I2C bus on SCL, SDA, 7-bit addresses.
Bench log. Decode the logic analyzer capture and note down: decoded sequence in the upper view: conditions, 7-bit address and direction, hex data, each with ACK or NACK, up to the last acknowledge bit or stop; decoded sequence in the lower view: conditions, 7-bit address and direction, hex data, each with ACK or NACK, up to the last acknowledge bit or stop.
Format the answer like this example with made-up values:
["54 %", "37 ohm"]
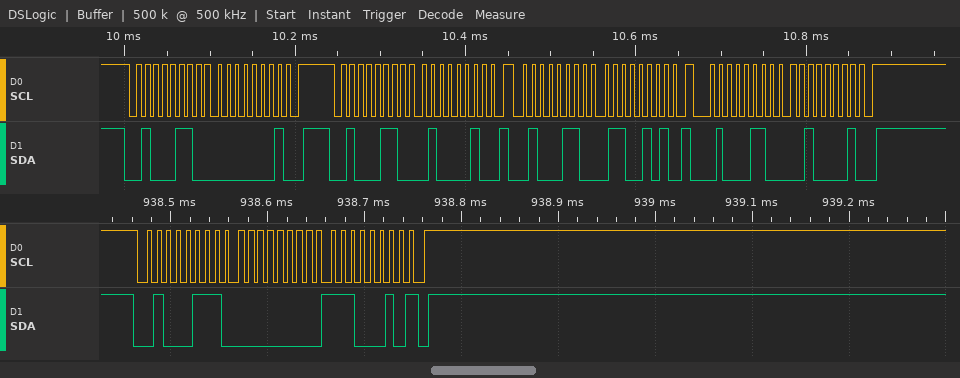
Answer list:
["start, address 23 write ACK, 01 ACK, stop, start, address 23 write ACK, 42 ACK, repeated start, address 23 write ACK, 65 ACK, repeated start, address 23 write ACK, 21 ACK, stop", "start, address 23 read ACK, 00 ACK, E2 NACK, stop"]
